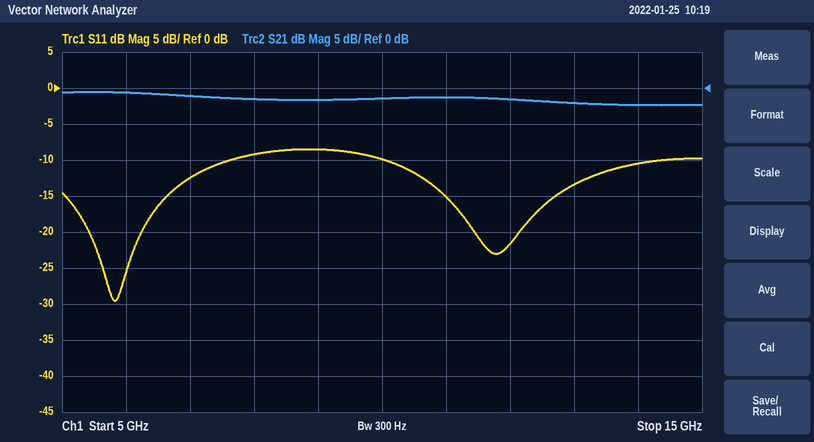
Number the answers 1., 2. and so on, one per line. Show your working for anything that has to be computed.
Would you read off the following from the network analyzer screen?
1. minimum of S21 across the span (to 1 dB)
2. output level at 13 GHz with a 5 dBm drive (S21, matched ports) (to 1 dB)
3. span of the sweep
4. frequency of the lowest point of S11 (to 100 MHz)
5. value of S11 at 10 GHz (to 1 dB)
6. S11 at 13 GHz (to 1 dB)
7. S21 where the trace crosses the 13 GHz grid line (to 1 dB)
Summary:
1. -2 dB
2. 5 dBm + (-2 dB) = 3 dBm
3. 10 GHz
4. 5.8 GHz
5. -10 dB
6. -13 dB
7. -2 dB
